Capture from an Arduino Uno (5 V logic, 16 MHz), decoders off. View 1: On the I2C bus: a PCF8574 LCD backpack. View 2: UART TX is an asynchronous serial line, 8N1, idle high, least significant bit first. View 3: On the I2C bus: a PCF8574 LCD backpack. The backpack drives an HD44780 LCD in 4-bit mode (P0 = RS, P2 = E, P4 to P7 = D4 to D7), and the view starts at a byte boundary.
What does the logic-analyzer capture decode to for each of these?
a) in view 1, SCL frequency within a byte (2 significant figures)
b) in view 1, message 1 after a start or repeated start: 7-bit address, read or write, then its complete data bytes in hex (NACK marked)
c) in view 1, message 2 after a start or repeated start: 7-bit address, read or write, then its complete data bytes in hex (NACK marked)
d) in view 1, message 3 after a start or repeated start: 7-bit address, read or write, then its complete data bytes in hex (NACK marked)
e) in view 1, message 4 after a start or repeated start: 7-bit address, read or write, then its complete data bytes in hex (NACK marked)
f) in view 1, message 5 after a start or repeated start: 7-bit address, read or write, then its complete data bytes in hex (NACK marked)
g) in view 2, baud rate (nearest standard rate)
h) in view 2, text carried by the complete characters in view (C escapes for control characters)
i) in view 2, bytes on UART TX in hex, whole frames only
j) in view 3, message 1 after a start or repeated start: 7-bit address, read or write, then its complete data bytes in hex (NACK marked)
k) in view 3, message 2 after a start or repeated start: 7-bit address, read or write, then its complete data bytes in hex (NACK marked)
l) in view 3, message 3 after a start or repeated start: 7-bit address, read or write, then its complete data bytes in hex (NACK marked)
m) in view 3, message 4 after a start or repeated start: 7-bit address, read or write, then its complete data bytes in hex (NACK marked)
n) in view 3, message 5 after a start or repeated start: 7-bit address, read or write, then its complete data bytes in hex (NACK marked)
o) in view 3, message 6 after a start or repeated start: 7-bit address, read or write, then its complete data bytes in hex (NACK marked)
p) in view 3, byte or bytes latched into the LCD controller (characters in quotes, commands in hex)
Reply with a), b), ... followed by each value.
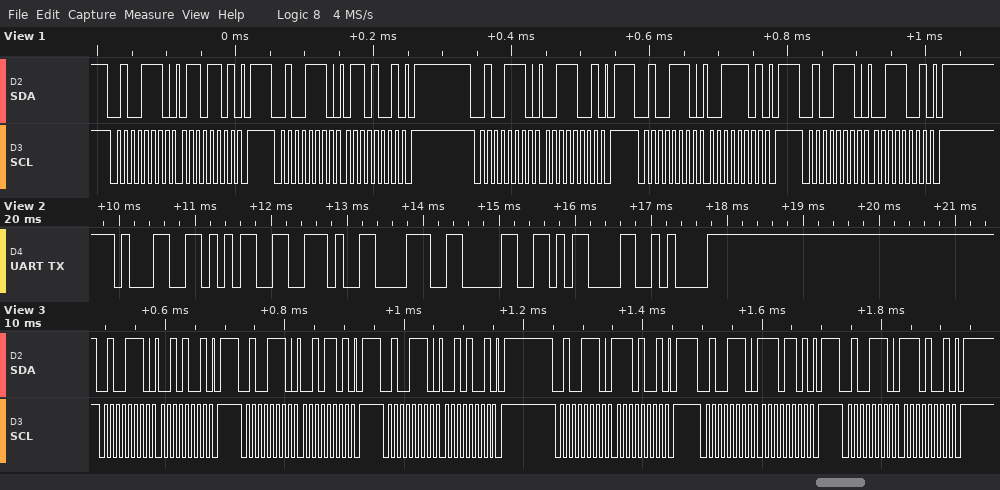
a) 100 kHz
b) 0x27 write: 6D
c) 0x27 write: 69
d) 0x27 write: 39
e) 0x27 write: 3D
f) 0x27 write: 39
g) 9600 baud
h) "15.80\r\n"
i) 31 35 2E 38 30 0D 0A
j) 0x27 write: 29
k) 0x27 write: 2D
l) 0x27 write: 29
m) 0x27 write: E9
n) 0x27 write: ED
o) 0x27 write: E9
p) '.'
